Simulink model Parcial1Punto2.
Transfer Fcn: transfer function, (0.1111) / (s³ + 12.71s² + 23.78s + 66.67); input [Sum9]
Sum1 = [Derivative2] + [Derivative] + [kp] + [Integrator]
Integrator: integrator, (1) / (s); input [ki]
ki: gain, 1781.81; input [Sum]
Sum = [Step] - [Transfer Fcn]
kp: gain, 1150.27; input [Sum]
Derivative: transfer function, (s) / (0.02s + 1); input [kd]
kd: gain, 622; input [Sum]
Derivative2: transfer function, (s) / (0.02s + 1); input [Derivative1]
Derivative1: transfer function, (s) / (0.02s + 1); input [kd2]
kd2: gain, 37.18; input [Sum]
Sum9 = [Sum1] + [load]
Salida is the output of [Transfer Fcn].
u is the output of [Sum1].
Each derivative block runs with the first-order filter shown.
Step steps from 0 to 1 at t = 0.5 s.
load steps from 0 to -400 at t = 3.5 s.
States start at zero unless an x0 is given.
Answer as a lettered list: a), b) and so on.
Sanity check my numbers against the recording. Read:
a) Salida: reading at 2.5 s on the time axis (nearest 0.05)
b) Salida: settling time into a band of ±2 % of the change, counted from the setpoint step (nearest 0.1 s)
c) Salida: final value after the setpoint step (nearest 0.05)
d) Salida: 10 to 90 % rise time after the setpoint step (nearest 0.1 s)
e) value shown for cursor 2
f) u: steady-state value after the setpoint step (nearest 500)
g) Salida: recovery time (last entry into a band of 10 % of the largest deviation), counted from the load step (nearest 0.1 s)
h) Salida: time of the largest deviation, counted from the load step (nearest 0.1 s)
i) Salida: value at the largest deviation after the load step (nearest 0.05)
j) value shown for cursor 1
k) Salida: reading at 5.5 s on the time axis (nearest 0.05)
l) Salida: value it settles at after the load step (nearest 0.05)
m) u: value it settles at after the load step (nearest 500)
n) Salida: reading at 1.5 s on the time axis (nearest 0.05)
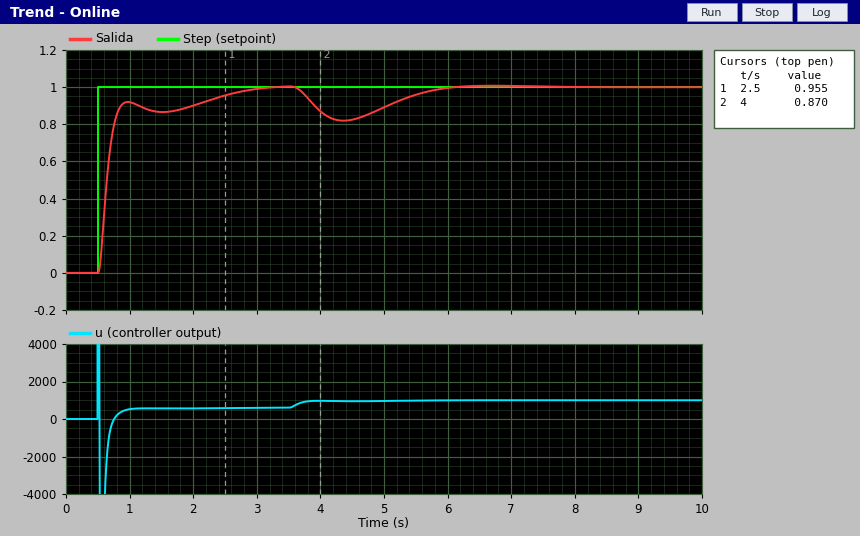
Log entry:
a) 0.95
b) 2.3 s
c) 1.00
d) 0.3 s
e) 0.870
f) 500
g) 2.3 s
h) 0.9 s
i) 0.80
j) 0.955
k) 0.95
l) 1.00
m) 1000
n) 0.85
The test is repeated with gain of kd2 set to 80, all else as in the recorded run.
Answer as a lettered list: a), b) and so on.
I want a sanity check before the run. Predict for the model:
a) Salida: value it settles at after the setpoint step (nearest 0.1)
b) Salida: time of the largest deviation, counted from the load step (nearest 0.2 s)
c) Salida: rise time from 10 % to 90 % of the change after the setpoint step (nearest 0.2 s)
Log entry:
a) 1.0
b) 1.0 s
c) 1.4 s
